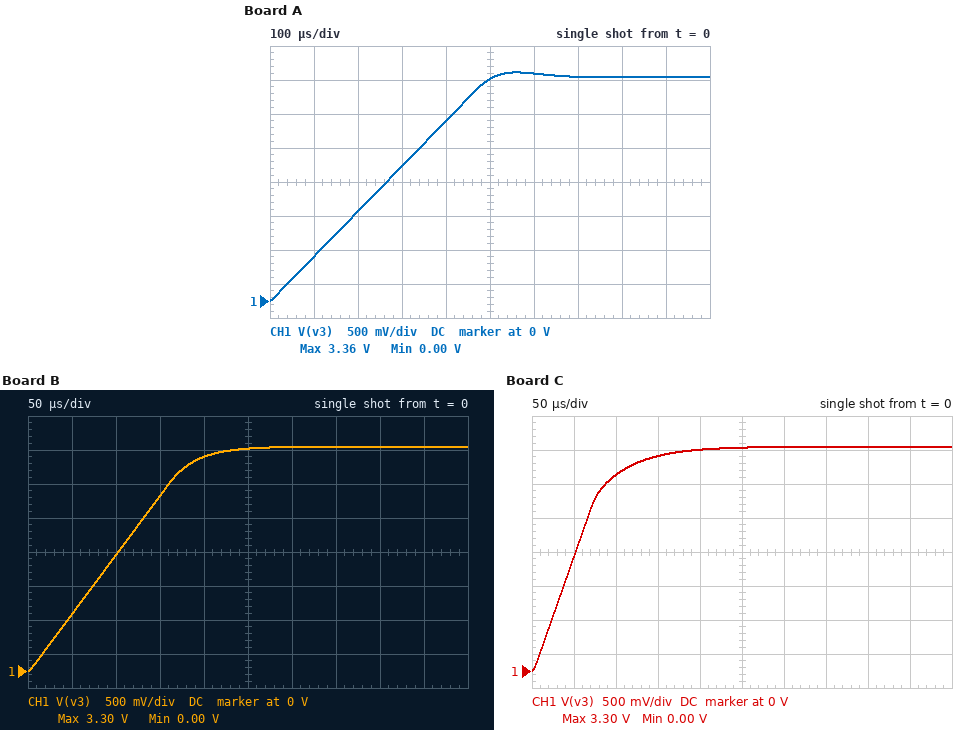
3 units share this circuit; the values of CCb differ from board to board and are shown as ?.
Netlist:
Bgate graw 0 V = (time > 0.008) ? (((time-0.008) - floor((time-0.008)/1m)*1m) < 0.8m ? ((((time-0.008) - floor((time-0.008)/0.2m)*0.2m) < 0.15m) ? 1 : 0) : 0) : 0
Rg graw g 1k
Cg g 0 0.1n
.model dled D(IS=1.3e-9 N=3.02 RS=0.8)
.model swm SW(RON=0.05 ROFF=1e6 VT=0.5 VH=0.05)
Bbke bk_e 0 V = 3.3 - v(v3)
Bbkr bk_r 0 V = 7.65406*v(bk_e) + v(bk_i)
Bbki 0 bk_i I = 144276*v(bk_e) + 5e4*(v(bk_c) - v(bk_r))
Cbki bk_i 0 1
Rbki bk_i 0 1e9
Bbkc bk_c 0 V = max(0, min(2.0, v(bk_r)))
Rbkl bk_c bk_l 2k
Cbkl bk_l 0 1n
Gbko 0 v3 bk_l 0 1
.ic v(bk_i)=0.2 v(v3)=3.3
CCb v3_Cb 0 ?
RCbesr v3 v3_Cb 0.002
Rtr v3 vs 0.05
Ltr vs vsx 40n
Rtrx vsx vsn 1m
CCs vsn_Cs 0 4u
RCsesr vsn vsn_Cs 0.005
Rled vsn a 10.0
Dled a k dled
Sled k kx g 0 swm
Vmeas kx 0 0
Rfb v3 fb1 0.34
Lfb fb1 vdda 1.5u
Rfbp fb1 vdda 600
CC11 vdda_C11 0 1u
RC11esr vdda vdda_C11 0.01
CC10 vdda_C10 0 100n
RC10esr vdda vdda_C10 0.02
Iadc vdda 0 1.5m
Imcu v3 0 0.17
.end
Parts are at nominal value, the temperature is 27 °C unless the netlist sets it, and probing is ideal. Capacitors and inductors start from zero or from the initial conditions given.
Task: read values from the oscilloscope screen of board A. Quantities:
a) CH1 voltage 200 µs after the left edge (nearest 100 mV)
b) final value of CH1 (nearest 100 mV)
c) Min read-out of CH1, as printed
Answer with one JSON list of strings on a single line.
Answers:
["1.3 V", "3.3 V", "0.00 V"]
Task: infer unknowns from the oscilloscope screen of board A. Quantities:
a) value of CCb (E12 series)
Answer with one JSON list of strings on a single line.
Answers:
["270 µF"]
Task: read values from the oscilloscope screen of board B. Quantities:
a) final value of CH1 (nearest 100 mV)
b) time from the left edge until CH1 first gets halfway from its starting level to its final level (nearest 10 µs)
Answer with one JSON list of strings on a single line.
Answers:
["3.3 V", "100 µs"]
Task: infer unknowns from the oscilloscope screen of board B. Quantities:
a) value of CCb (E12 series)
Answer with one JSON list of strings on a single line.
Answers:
["100 µF"]
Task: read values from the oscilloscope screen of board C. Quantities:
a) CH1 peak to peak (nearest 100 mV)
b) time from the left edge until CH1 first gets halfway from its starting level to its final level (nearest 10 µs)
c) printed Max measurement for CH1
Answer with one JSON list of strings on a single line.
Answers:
["3.3 V", "50 µs", "3.30 V"]
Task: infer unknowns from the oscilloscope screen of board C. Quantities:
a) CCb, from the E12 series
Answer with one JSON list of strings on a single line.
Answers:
["47 µF"]
